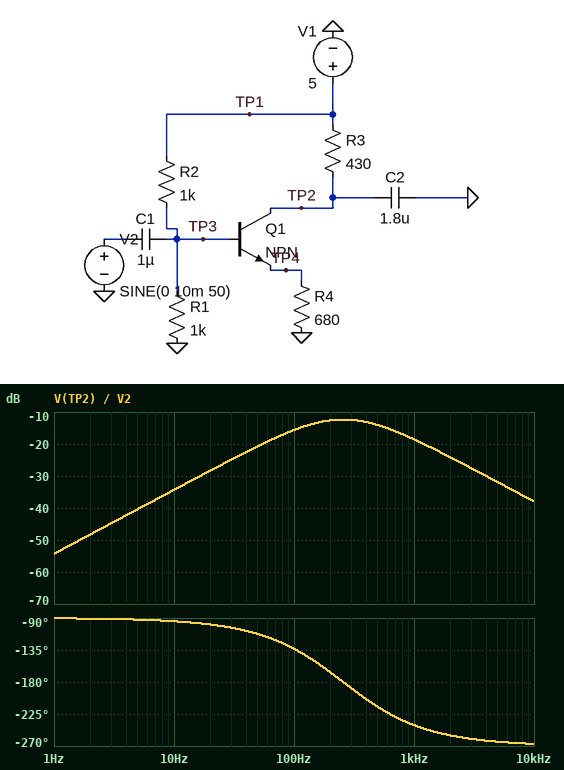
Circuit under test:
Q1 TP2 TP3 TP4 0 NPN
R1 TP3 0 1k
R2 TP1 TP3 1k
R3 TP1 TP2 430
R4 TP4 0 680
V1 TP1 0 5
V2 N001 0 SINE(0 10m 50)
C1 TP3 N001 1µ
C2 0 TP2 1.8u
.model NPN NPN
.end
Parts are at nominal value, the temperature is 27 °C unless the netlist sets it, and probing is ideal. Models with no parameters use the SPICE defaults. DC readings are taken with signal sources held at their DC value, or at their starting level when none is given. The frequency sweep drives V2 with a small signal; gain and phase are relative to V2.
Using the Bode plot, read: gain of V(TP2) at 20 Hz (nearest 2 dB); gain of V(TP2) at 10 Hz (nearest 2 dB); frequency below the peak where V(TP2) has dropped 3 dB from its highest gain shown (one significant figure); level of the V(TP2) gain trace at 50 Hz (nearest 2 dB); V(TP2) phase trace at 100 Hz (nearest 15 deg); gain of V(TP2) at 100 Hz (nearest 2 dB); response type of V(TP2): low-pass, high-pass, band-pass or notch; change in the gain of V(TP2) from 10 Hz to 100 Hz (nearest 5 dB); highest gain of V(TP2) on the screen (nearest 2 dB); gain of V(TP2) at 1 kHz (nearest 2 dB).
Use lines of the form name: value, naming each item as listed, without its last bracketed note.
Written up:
gain of V(TP2) at 20 Hz: -28 dB
gain of V(TP2) at 10 Hz: -34 dB
frequency below the peak where V(TP2) has dropped 3 dB from its highest gain shown: 100 Hz
level of the V(TP2) gain trace at 50 Hz: -20 dB
V(TP2) phase trace at 100 Hz: -135 deg
gain of V(TP2) at 100 Hz: -16 dB
response type of V(TP2): low-pass, high-pass, band-pass or notch: band-pass
change in the gain of V(TP2) from 10 Hz to 100 Hz: 20 dB
highest gain of V(TP2) on the screen: -12 dB
gain of V(TP2) at 1 kHz: -18 dB
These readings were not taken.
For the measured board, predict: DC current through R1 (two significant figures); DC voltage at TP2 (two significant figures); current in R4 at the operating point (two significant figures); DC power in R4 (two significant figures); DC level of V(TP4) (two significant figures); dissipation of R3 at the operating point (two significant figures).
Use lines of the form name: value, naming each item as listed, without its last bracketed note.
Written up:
DC current through R1: 2.5 mA
DC voltage at TP2: 3.9 V
current in R4 at the operating point: 2.5 mA
DC power in R4: 4.2 mW
DC level of V(TP4): 1.7 V
dissipation of R3 at the operating point: 2.6 mW
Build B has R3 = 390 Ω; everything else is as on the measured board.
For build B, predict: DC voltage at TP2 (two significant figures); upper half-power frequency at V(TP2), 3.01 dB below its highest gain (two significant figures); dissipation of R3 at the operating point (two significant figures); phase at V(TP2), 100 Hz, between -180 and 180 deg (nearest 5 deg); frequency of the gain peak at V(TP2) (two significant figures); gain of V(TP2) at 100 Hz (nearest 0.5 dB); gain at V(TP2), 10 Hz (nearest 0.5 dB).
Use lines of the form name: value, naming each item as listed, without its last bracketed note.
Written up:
DC voltage at TP2: 4.0 V
upper half-power frequency at V(TP2), 3.01 dB below its highest gain: 660 Hz
dissipation of R3 at the operating point: 2.4 mW
phase at V(TP2), 100 Hz, between -180 and 180 deg: -130 deg
frequency of the gain peak at V(TP2): 270 Hz
gain of V(TP2) at 100 Hz: -16.5 dB
gain at V(TP2), 10 Hz: -35.0 dB
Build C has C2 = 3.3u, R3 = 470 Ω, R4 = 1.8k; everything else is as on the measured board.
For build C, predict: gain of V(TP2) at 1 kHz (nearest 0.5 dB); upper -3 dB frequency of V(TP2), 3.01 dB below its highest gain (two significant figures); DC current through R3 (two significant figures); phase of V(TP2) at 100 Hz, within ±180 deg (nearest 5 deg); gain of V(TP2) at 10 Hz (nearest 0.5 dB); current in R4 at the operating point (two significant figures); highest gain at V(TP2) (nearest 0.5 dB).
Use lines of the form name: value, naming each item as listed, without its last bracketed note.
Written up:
gain of V(TP2) at 1 kHz: -32.0 dB
upper -3 dB frequency of V(TP2), 3.01 dB below its highest gain: 490 Hz
DC current through R3: 950 µA
phase of V(TP2) at 100 Hz, within ±180 deg: -150 deg
gain of V(TP2) at 10 Hz: -42.0 dB
current in R4 at the operating point: 960 µA
highest gain at V(TP2): -24.0 dB
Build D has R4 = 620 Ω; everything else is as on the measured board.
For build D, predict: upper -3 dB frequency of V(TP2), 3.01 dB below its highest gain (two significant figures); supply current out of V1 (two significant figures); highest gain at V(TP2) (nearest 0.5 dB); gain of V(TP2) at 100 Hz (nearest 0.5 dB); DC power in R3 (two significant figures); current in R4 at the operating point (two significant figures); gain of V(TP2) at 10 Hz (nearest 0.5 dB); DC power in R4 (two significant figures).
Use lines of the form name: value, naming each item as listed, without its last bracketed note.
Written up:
upper -3 dB frequency of V(TP2), 3.01 dB below its highest gain: 630 Hz
supply current out of V1: 5.2 mA
highest gain at V(TP2): -11.5 dB
gain of V(TP2) at 100 Hz: -15.0 dB
DC power in R3: 3.1 mW
current in R4 at the operating point: 2.7 mA
gain of V(TP2) at 10 Hz: -33.5 dB
DC power in R4: 4.6 mW
